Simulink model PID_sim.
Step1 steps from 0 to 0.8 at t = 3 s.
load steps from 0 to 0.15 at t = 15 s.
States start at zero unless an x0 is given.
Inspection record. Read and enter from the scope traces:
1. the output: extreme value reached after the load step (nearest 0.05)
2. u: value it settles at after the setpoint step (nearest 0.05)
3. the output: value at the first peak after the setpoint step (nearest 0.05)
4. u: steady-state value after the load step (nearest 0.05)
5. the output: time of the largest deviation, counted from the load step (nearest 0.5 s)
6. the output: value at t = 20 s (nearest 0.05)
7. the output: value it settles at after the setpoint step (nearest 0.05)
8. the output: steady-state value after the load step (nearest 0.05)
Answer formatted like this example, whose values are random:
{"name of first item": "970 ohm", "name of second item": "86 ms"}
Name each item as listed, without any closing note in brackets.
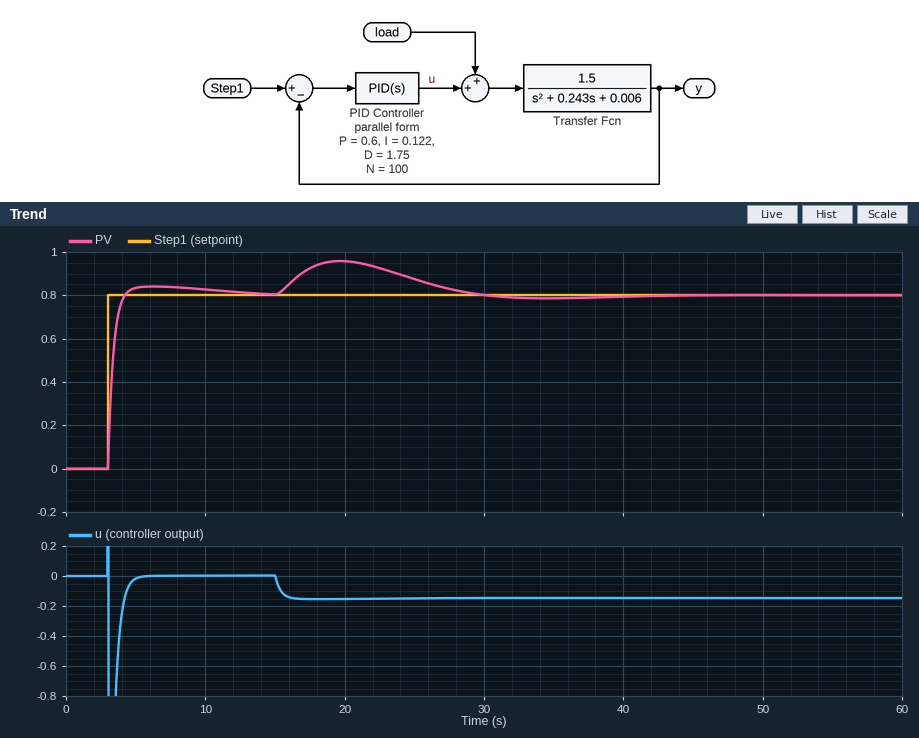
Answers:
{"the output: extreme value reached after the load step": "0.95", "u: value it settles at after the setpoint step": "0.00", "the output: value at the first peak after the setpoint step": "0.85", "u: steady-state value after the load step": "-0.15", "the output: time of the largest deviation, counted from the load step": "4.5 s", "the output: value at t = 20 s": "0.95", "the output: value it settles at after the setpoint step": "0.80", "the output: steady-state value after the load step": "0.80"}
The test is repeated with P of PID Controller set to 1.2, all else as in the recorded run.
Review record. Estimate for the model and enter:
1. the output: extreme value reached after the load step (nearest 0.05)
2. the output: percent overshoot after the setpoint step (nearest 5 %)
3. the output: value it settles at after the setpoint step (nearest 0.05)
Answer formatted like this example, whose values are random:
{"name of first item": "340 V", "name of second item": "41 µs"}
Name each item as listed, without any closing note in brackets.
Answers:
{"the output: extreme value reached after the load step": "0.90", "the output: percent overshoot after the setpoint step": "10 %", "the output: value it settles at after the setpoint step": "0.80"}
